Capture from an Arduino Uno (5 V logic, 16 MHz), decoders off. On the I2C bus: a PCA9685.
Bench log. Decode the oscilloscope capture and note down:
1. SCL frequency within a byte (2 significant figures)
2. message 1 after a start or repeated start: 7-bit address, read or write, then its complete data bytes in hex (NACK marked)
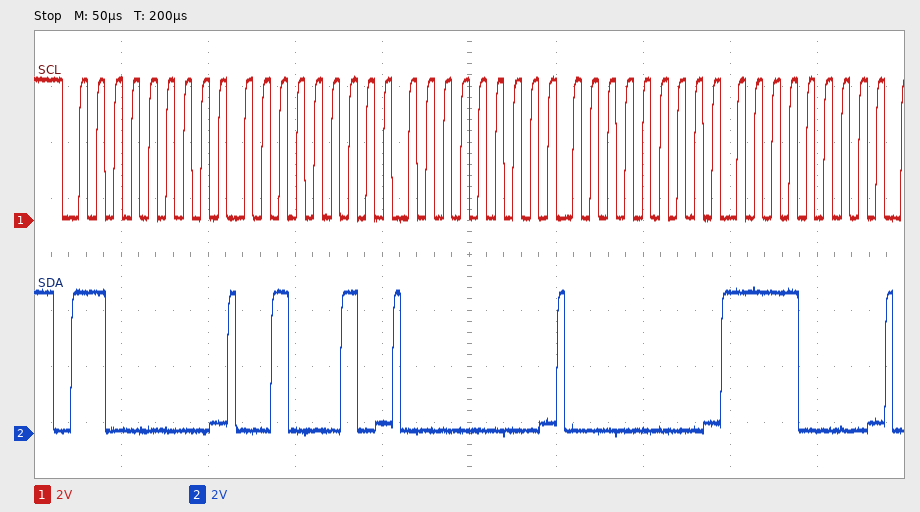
100 kHz
0x60 write: 22 00 00 F0
